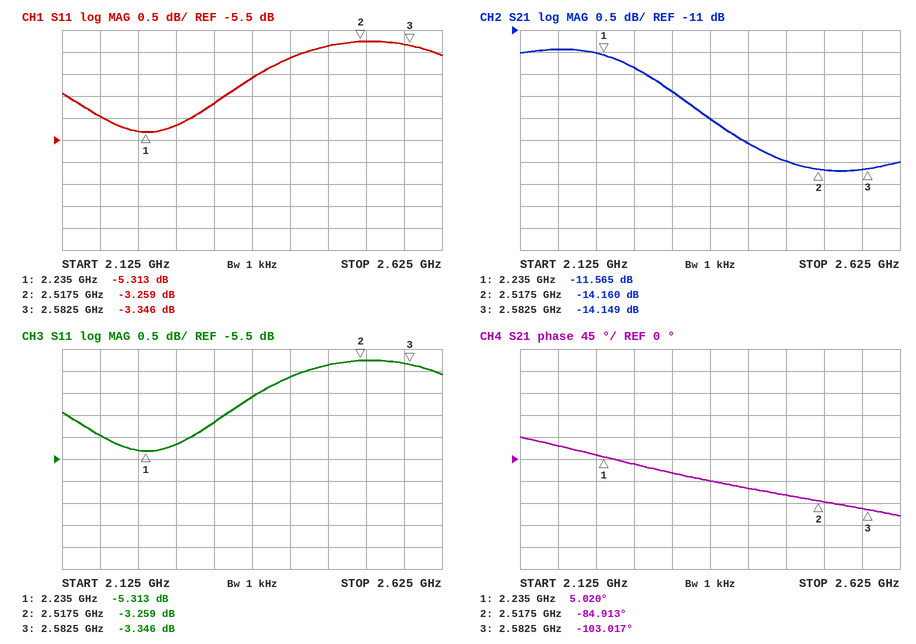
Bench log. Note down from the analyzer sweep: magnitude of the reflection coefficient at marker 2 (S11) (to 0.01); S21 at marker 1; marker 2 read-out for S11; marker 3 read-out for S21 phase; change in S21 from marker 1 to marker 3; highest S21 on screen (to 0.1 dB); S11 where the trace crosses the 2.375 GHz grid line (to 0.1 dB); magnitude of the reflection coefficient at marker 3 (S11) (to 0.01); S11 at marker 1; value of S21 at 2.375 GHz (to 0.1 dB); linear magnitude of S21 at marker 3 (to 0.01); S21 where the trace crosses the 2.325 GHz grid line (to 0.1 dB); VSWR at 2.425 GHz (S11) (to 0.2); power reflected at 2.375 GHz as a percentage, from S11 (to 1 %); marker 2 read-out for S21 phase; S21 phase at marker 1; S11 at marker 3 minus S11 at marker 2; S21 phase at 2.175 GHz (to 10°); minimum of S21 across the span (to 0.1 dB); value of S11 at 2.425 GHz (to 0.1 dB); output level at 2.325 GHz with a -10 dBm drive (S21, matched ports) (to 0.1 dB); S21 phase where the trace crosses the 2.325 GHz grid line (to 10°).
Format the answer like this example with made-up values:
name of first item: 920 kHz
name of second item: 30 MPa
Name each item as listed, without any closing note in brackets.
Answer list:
magnitude of the reflection coefficient at marker 2 (S11): 0.69
S21 at marker 1: -11.565 dB
marker 2 read-out for S11: -3.259 dB
marker 3 read-out for S21 phase: -103.017°
change in S21 from marker 1 to marker 3: -2.584 dB
highest S21 on screen: -11.4 dB
S11 where the trace crosses the 2.375 GHz grid line: -4.1 dB
magnitude of the reflection coefficient at marker 3 (S11): 0.68
S11 at marker 1: -5.313 dB
value of S21 at 2.375 GHz: -13.0 dB
linear magnitude of S21 at marker 3: 0.20
S21 where the trace crosses the 2.325 GHz grid line: -12.4 dB
VSWR at 2.425 GHz (S11): 4.8
power reflected at 2.375 GHz as a percentage, from S11: 39 %
marker 2 read-out for S21 phase: -84.913°
S21 phase at marker 1: 5.020°
S11 at marker 3 minus S11 at marker 2: -0.087 dB
S21 phase at 2.175 GHz: 30°
minimum of S21 across the span: -14.2 dB
value of S11 at 2.425 GHz: -3.6 dB
output level at 2.325 GHz with a -10 dBm drive (S21, matched ports): -22.4 dBm
S21 phase where the trace crosses the 2.325 GHz grid line: -30°
